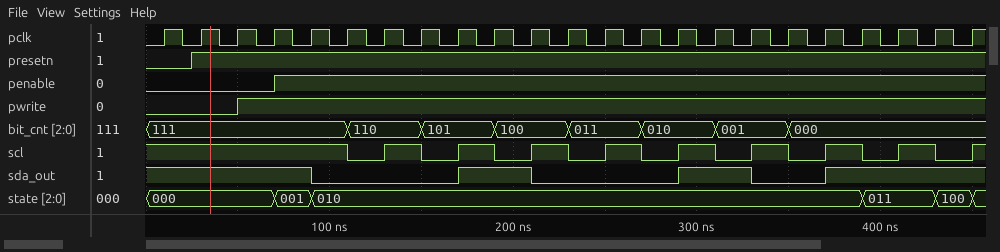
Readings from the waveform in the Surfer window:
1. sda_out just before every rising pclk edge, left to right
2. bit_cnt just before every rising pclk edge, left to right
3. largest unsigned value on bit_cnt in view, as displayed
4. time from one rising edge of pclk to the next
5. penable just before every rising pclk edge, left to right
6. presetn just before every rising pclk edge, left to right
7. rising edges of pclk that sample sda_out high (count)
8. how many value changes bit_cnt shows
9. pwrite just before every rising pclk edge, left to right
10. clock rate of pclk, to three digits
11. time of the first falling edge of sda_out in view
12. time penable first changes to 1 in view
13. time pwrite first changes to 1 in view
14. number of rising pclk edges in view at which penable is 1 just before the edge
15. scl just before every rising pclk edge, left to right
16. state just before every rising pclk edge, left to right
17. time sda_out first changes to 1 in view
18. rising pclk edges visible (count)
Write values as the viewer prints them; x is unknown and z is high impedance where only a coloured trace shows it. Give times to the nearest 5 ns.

1 1 1 1 1 0 0 0 0 1 1 0 0 0 0 1 1 0 0 1 1 1 1
111, 111, 111, 111, 111, 111, 110, 110, 101, 101, 100, 100, 011, 011, 010, 010, 001, 001, 000, 000, 000, 000, 000
111
20 ns
0 0 0 0 1 1 1 1 1 1 1 1 1 1 1 1 1 1 1 1 1 1 1
0 1 1 1 1 1 1 1 1 1 1 1 1 1 1 1 1 1 1 1 1 1 1
13
7
0 0 0 1 1 1 1 1 1 1 1 1 1 1 1 1 1 1 1 1 1 1 1
50.0 MHz
90 ns
70 ns
50 ns
19
1 1 1 1 1 1 0 1 0 1 0 1 0 1 0 1 0 1 0 1 0 1 0
000, 000, 000, 000, 001, 010, 010, 010, 010, 010, 010, 010, 010, 010, 010, 010, 010, 010, 010, 010, 011, 011, 100
170 ns
23
